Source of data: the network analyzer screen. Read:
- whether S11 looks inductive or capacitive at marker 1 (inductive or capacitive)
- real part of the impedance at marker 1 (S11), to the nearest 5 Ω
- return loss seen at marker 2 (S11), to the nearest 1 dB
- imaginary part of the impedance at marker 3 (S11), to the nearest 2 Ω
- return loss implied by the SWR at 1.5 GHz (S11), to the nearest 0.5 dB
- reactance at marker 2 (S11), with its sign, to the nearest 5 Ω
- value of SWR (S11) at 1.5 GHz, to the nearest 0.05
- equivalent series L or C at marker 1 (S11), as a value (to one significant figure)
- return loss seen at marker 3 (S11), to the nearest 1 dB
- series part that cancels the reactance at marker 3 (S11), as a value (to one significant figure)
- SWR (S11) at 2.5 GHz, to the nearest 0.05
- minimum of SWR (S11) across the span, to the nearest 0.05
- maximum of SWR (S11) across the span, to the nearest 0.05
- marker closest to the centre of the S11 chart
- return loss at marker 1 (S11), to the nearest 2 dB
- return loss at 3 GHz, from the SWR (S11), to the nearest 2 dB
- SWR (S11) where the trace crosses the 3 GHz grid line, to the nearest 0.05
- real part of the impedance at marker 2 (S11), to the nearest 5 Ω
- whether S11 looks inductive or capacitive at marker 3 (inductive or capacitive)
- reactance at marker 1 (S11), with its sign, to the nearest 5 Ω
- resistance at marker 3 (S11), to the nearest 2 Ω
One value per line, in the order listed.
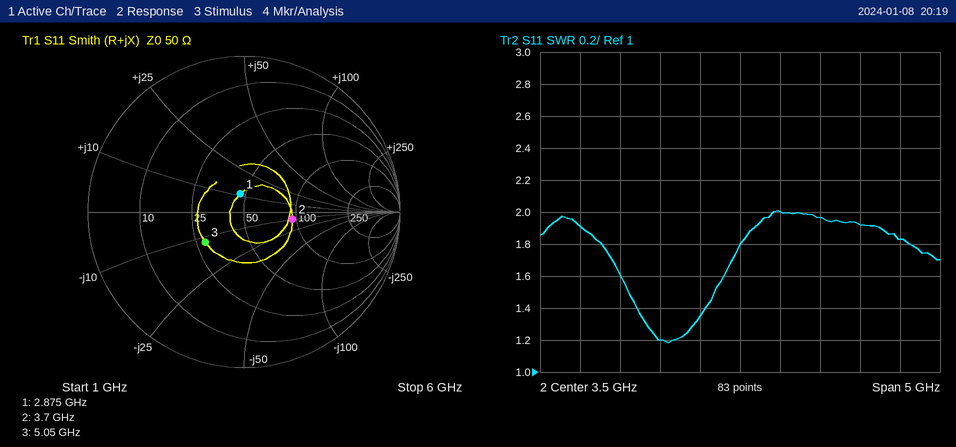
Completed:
inductive
45 Ω
10 dB
-12 Ω
10.0 dB
-10 Ω
1.90
600 pH
10 dB
400 pH
1.20
1.20
2.00
marker 1
18 dB
16 dB
1.35
95 Ω
capacitive
+10 Ω
28 Ω
